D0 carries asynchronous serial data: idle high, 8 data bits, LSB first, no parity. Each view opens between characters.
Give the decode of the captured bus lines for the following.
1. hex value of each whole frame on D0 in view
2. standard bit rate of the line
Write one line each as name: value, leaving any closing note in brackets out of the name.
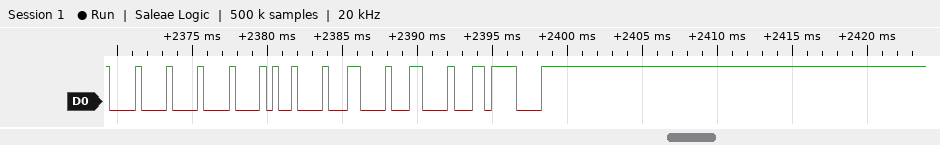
hex value of each whole frame on D0 in view: 08, 08, 28, 88, 88, 88, 0F
standard bit rate of the line: 2400 baud
